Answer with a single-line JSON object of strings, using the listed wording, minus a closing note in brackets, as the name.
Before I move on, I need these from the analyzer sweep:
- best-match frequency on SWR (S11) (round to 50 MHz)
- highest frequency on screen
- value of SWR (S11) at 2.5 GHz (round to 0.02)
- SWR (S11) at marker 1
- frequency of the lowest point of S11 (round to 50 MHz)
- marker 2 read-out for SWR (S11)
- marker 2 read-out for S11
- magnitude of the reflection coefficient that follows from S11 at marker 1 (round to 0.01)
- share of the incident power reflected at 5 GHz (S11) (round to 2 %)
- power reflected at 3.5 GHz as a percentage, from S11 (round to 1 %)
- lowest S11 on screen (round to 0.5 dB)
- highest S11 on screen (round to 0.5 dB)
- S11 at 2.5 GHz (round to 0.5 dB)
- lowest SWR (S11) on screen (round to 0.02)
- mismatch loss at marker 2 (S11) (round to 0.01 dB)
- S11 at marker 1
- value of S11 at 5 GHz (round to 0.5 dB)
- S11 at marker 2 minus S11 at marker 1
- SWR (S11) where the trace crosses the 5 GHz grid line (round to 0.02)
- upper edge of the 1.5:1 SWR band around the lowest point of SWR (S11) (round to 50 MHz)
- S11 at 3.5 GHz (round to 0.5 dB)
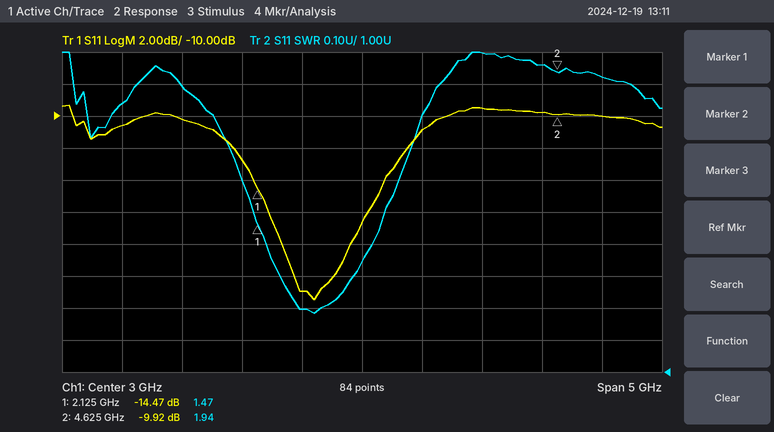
{"best-match frequency on SWR (S11)": "2.60 GHz", "highest frequency on screen": "5.5 GHz", "value of SWR (S11) at 2.5 GHz": "1.20", "SWR (S11) at marker 1": "1.47", "frequency of the lowest point of S11": "2.60 GHz", "marker 2 read-out for SWR": "1.94", "marker 2 read-out for S11": "-9.92 dB", "magnitude of the reflection coefficient that follows from S11 at marker 1": "0.19", "share of the incident power reflected at 5 GHz (S11)": "10 %", "power reflected at 3.5 GHz as a percentage, from S11": "8 %", "lowest S11 on screen": "-21.5 dB", "highest S11 on screen": "-9.5 dB", "S11 at 2.5 GHz": "-21.0 dB", "lowest SWR (S11) on screen": "1.18", "mismatch loss at marker 2 (S11)": "0.47 dB", "S11 at marker 1": "-14.47 dB", "value of S11 at 5 GHz": "-10.0 dB", "S11 at marker 2 minus S11 at marker 1": "4.55 dB", "SWR (S11) where the trace crosses the 5 GHz grid line": "1.92", "upper edge of the 1.5:1 SWR band around the lowest point of SWR (S11)": "3.20 GHz", "S11 at 3.5 GHz": "-11.0 dB"}
